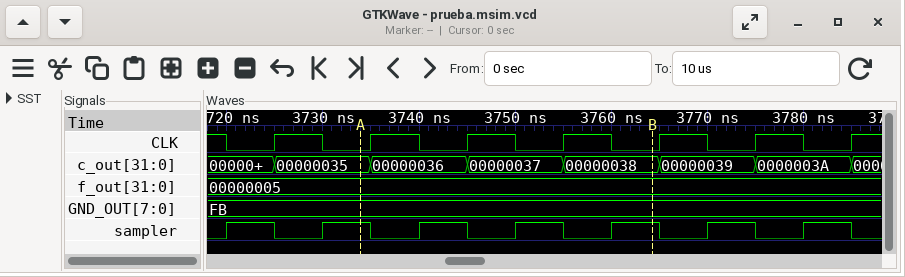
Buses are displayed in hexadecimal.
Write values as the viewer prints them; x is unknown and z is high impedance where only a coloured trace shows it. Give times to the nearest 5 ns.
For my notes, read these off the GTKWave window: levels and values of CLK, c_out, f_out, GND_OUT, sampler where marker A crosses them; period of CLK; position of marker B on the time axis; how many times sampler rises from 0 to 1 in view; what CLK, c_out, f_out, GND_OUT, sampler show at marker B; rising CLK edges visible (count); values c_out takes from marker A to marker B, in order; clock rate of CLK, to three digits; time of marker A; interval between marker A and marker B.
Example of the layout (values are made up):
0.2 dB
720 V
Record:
CLK=0, c_out=00000035, f_out=00000005, GND_OUT=FB, sampler=1
10 ns
3765 ns
7
CLK=0, c_out=00000038, f_out=00000005, GND_OUT=FB, sampler=1
7
00000035, 00000036, 00000037, 00000038
100 MHz
3735 ns
30 ns
